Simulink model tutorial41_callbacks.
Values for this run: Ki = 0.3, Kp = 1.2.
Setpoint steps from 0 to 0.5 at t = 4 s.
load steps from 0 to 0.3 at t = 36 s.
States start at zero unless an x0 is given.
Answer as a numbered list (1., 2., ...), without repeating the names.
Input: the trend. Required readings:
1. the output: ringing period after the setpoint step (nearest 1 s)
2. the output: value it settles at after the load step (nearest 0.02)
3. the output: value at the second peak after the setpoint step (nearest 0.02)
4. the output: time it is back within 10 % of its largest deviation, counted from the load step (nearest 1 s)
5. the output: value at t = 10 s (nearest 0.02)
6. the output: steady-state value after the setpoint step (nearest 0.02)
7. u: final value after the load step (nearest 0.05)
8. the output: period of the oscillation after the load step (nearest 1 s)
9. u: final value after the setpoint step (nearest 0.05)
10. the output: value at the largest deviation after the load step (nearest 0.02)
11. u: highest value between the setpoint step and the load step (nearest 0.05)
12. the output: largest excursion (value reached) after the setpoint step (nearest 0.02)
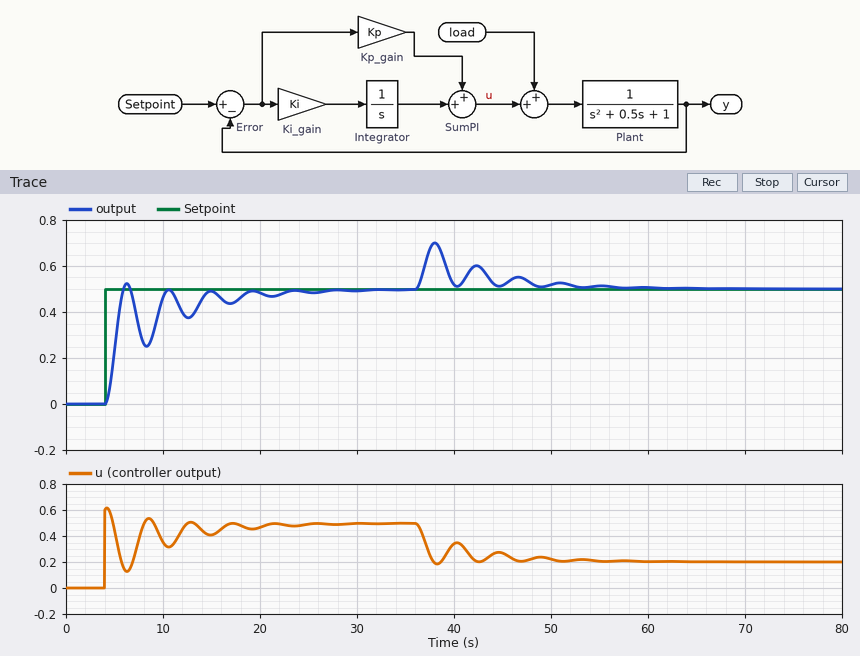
1. 4 s
2. 0.50
3. 0.50
4. 16 s
5. 0.46
6. 0.50
7. 0.20
8. 4 s
9. 0.50
10. 0.70
11. 0.60
12. 0.52
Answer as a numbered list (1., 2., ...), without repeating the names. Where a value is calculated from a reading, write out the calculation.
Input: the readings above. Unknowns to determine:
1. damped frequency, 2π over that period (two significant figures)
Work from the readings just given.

1. 2π / 4 = 1.6 rad/s
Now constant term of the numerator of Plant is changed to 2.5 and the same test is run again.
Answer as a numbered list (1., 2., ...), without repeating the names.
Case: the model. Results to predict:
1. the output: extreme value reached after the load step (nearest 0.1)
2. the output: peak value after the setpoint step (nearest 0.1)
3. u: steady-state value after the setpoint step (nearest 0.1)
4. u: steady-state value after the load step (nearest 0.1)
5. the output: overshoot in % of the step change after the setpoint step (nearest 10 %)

1. 0.8
2. 0.7
3. 0.2
4. -0.1
5. 40 %
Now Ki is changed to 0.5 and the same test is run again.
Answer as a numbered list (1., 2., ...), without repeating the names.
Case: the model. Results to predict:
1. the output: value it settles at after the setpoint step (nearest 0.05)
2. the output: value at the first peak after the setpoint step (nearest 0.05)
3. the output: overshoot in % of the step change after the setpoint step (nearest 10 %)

1. 0.50
2. 0.60
3. 20 %
